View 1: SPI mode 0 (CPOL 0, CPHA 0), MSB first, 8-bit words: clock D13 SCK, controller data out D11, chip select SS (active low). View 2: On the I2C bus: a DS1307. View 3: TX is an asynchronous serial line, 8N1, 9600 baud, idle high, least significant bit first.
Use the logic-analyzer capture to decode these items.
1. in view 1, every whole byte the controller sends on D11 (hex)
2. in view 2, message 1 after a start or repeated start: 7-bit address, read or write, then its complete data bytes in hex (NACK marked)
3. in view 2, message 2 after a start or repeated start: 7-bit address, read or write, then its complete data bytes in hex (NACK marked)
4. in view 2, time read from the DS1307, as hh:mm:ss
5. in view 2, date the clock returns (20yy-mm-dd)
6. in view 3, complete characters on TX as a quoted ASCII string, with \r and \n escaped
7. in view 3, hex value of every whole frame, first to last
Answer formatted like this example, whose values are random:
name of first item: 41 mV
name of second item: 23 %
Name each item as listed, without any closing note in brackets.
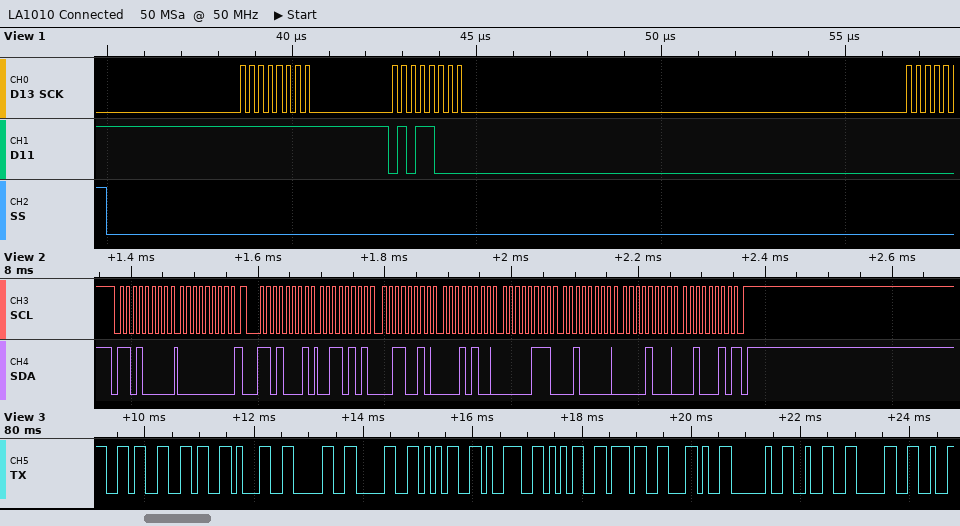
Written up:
in view 1, every whole byte the controller sends on D11: FF 58
in view 2, message 1 after a start or repeated start: 7-bit address, read or write, then its complete data bytes in hex: 0x68 write: 00
in view 2, message 2 after a start or repeated start: 7-bit address, read or write, then its complete data bytes in hex: 0x68 read: 35 32 14 07 20 08 22 NACK
in view 2, time read from the DS1307, as hh:mm:ss: 14:32:35
in view 2, date the clock returns: 2022-08-20
in view 3, complete characters on TX as a quoted ASCII string, with \r and \n escaped: "661005957, 20"
in view 3, hex value of every whole frame, first to last: 36 36 31 30 30 35 39 35 37 2C 20 32 30
